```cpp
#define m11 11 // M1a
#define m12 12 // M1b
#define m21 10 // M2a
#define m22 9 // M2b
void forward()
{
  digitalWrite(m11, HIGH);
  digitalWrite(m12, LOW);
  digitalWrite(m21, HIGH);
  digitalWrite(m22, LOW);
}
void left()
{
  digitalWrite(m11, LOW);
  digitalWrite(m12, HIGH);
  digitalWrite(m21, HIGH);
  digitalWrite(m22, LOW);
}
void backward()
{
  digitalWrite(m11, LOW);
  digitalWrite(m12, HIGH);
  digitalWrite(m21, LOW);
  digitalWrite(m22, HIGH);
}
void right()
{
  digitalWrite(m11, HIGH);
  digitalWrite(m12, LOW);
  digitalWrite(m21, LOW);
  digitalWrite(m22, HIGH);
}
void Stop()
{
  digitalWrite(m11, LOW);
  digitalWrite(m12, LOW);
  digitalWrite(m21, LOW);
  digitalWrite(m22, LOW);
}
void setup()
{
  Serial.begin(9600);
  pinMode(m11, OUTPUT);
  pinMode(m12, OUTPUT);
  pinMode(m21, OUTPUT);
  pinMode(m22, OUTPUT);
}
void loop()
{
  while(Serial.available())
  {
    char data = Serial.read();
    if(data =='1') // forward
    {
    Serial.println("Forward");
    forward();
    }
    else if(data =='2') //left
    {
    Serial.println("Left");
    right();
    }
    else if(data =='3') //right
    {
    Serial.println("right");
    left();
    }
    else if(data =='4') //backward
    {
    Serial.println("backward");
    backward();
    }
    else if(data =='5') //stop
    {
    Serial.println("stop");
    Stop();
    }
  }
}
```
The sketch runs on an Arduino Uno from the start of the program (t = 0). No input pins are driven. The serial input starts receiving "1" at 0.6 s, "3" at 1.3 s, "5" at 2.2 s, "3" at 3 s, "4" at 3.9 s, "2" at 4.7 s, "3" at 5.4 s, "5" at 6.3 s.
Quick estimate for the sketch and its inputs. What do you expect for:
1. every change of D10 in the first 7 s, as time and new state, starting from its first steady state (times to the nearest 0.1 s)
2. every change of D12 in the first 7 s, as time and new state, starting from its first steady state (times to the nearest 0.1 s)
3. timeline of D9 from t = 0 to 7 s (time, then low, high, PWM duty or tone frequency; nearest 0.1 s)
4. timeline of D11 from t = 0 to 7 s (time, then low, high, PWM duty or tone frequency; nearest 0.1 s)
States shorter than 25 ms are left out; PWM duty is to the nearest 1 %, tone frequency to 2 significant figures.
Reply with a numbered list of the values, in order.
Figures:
1. 0 s low; 0.6 s high; 2.2 s low; 3 s high; 3.9 s low; 5.4 s high; 6.3 s low
2. 0 s low; 1.3 s high; 2.2 s low; 3 s high; 4.7 s low; 5.4 s high; 6.3 s low
3. 0 s low; 3.9 s high; 5.4 s low
4. 0 s low; 0.6 s high; 1.3 s low; 4.7 s high; 5.4 s low
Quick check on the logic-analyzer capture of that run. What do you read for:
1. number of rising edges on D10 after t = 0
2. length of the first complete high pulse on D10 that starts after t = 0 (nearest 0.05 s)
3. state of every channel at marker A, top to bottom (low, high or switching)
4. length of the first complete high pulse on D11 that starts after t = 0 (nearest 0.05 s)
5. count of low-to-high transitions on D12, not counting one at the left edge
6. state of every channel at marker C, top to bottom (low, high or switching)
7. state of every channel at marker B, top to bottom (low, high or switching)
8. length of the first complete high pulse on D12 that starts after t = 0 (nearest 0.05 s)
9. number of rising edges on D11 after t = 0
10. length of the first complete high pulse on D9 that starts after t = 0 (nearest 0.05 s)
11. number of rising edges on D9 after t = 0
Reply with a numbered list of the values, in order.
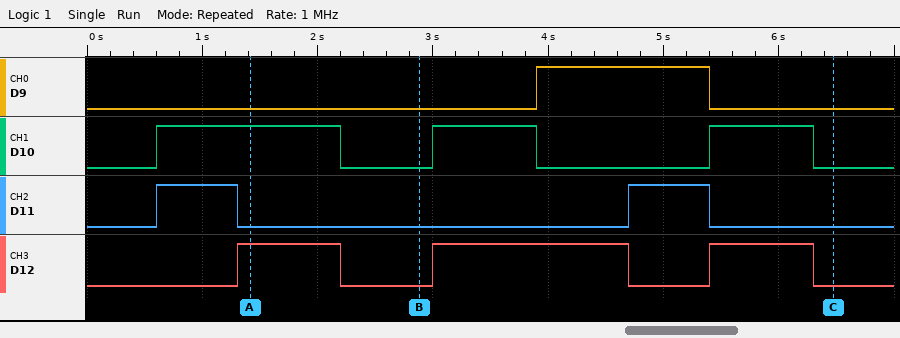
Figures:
1. 3
2. 1.60 s
3. D9 low, D10 high, D11 low, D12 high
4. 0.70 s
5. 3
6. D9 low, D10 low, D11 low, D12 low
7. D9 low, D10 low, D11 low, D12 low
8. 0.90 s
9. 2
10. 1.50 s
11. 1
